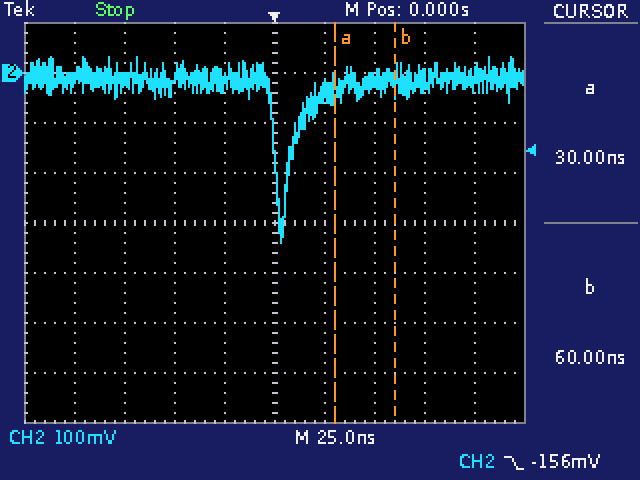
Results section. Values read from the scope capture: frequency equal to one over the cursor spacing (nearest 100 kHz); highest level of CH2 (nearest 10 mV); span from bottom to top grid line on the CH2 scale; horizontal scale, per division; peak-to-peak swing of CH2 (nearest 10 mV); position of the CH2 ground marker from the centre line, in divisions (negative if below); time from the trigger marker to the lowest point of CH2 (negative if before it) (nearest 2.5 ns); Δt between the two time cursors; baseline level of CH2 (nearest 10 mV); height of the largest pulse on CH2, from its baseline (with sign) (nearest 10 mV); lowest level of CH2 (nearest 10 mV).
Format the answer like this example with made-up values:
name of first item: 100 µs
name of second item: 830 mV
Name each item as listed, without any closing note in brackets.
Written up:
frequency equal to one over the cursor spacing: 33.3 MHz
highest level of CH2: 30 mV
span from bottom to top grid line on the CH2 scale: 800 mV
horizontal scale, per division: 25 ns
peak-to-peak swing of CH2: 370 mV
position of the CH2 ground marker from the centre line, in divisions: +3.0 div
time from the trigger marker to the lowest point of CH2 (negative if before it): +2.5 ns
Δt between the two time cursors: 30.0 ns
baseline level of CH2: -10 mV
height of the largest pulse on CH2, from its baseline (with sign): -330 mV
lowest level of CH2: -340 mV
